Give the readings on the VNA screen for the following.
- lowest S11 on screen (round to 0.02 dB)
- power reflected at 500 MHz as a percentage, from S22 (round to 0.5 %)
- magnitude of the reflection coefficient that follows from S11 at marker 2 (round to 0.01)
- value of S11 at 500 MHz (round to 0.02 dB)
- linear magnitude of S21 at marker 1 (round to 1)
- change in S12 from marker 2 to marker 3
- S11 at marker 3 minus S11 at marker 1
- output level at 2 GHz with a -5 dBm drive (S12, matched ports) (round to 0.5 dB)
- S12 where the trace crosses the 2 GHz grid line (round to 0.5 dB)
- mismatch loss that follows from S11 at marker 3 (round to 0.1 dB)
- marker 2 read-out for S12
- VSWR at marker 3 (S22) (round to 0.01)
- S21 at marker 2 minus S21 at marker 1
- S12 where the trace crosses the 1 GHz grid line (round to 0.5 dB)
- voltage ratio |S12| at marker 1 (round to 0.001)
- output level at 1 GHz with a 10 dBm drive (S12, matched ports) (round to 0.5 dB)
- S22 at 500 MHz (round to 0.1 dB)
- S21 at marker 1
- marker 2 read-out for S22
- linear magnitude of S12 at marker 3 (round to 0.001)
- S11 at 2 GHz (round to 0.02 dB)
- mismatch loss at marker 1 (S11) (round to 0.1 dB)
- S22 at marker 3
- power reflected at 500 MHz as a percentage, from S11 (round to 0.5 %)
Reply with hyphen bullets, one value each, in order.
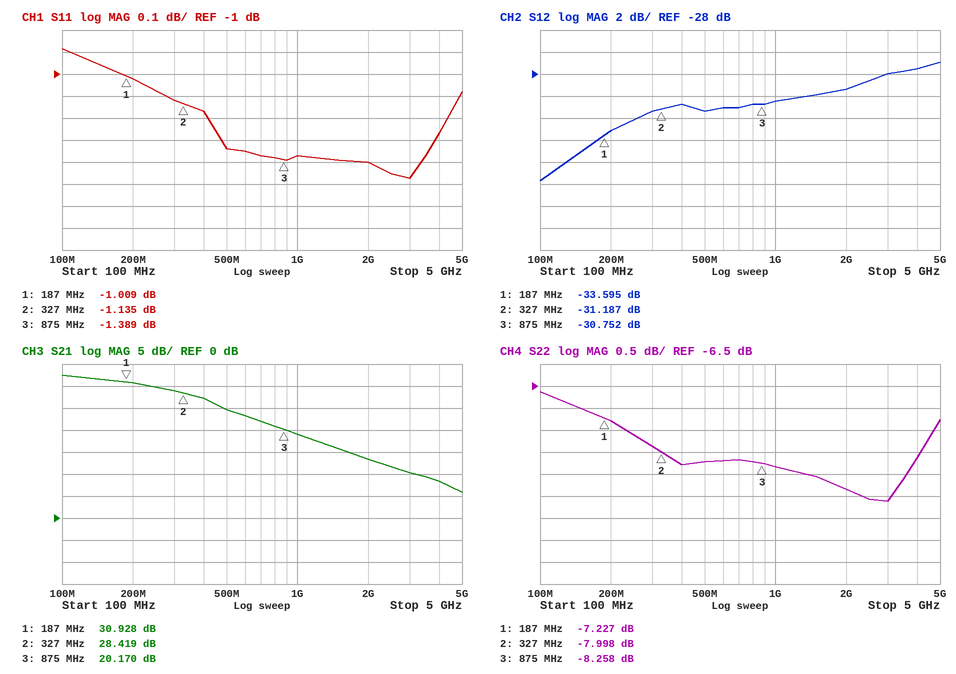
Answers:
- -1.48 dB
- 15.0 %
- 0.88
- -1.34 dB
- 35
- 0.435 dB
- -0.380 dB
- -34.5 dBm
- -29.5 dB
- 5.6 dB
- -31.187 dB
- 2.26
- -2.509 dB
- -30.5 dB
- 0.021
- -20.5 dBm
- -8.2 dB
- 30.928 dB
- -7.998 dB
- 0.029
- -1.40 dB
- 6.8 dB
- -8.258 dB
- 73.5 %
